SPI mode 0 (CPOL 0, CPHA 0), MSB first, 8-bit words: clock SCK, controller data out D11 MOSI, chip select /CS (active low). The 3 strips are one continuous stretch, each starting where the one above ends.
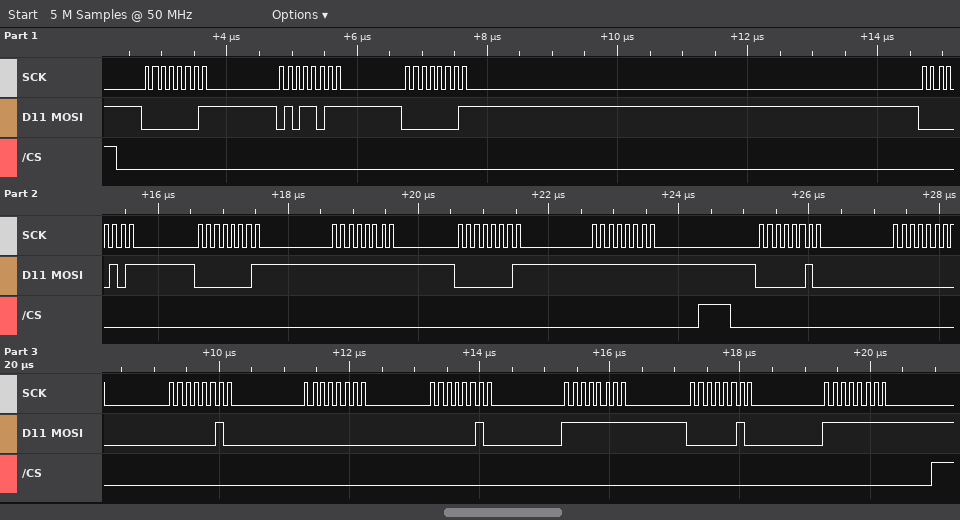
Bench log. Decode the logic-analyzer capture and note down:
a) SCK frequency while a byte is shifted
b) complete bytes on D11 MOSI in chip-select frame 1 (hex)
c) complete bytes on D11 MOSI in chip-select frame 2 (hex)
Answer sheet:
8 MHz
0x01 0x5B 0x01 0x05 0x01 0xFF 0x01 0xFF
0x02 0x00 0x02 0x00 0x02 0xFF 0x02 0xFF
